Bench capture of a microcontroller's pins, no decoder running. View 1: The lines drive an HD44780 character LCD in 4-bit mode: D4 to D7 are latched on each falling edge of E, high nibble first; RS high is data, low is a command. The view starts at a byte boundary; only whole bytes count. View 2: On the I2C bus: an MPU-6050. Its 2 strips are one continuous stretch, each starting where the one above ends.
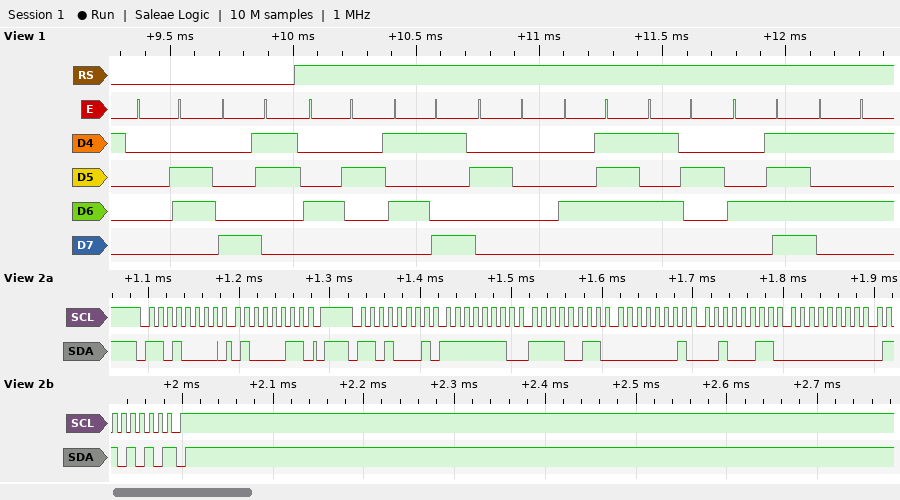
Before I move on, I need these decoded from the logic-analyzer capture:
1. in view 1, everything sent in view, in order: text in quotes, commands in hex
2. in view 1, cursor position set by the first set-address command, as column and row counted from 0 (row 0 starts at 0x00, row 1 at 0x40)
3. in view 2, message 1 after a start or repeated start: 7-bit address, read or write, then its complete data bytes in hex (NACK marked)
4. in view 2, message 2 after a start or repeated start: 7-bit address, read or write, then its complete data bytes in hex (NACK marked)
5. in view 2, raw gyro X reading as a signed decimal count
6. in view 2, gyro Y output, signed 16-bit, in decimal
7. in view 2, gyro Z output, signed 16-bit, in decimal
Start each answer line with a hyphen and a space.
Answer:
- 0x06 0x83 "BY GROU"
- column 3, row 0
- 0x68 write: 43
- 0x68 read: FE F3 01 23 00 6A NACK
- -269
- 291
- 106
